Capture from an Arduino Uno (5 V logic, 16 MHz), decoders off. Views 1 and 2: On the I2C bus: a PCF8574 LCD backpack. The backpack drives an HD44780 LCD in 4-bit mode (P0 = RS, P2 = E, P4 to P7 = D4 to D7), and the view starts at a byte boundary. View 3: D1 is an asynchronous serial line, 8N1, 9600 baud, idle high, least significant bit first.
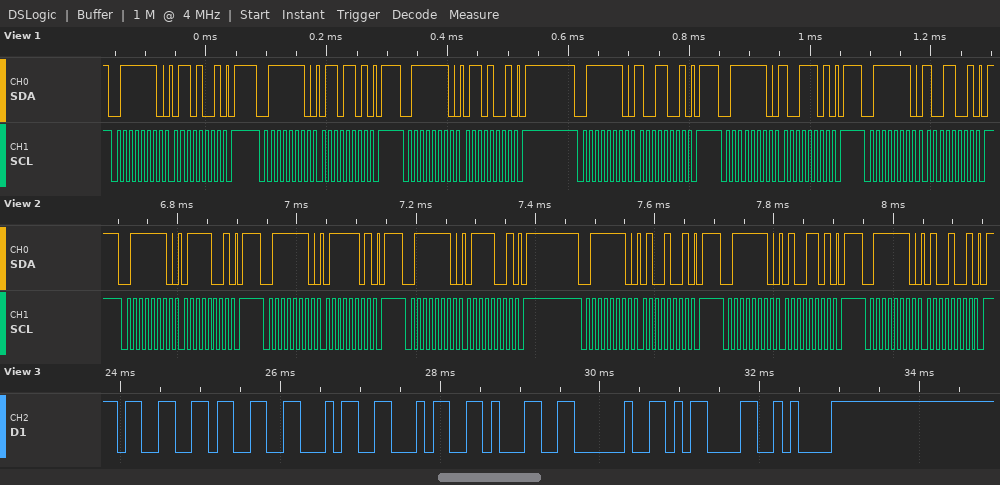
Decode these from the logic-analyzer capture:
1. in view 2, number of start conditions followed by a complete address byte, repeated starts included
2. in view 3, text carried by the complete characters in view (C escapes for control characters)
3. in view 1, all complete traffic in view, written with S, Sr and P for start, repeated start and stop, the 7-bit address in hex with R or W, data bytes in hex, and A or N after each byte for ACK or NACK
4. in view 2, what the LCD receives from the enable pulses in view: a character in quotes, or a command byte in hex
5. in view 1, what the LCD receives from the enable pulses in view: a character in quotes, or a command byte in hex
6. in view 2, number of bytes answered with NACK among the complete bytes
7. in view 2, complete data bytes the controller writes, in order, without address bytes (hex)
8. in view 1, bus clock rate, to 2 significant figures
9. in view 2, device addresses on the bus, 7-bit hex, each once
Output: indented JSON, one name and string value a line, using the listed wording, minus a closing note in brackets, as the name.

{
  "in view 2, number of start conditions followed by a complete address byte, repeated starts included": "6",
  "in view 3, text carried by the complete characters in view": "\"33441 \\r\\n\"",
  "in view 1, all complete traffic in view, written with S, Sr and P for start, repeated start and stop, the 7-bit address in hex with R or W, data bytes in hex, and A or N after each byte for ACK or NACK": "S 3FW A 69 A P S 3FW A 6D A P S 3FW A 69 A P S 3FW A 99 A P S 3FW A 9D A P S 3FW A 99 A P",
  "in view 2, what the LCD receives from the enable pulses in view: a character in quotes, or a command byte in hex": "'t'",
  "in view 1, what the LCD receives from the enable pulses in view: a character in quotes, or a command byte in hex": "'i'",
  "in view 2, number of bytes answered with NACK among the complete bytes": "0",
  "in view 2, complete data bytes the controller writes, in order, without address bytes": "79 7D 79 49 4D 49",
  "in view 1, bus clock rate, to 2 significant figures": "100 kHz",
  "in view 2, device addresses on the bus, 7-bit hex, each once": "0x3F"
}
